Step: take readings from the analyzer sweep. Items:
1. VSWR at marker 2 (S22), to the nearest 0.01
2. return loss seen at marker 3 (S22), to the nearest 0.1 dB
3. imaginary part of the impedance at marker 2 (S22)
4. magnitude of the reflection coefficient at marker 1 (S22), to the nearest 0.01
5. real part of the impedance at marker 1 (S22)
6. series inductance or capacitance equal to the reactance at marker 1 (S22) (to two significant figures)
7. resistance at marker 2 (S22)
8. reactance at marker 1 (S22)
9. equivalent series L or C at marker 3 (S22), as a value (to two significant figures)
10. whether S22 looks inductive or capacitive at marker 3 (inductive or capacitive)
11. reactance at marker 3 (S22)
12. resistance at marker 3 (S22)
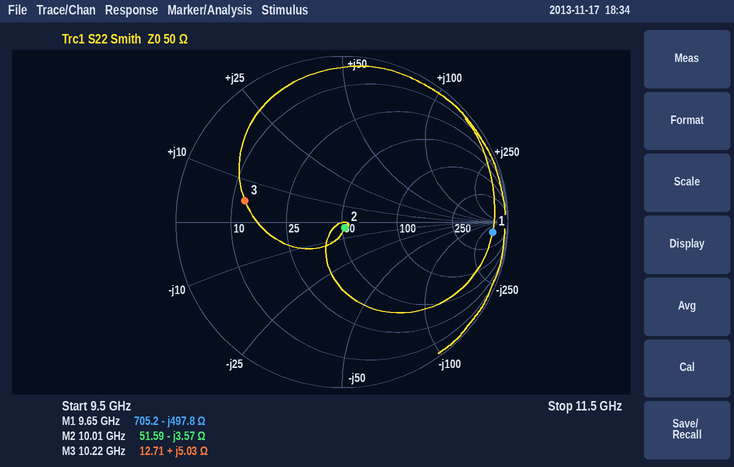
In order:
1.08
4.5 dB
-3.57 Ω
0.91
705.2 Ω
33 fF
51.59 Ω
-497.8 Ω
78 pH
inductive
+5.03 Ω
12.71 Ω
